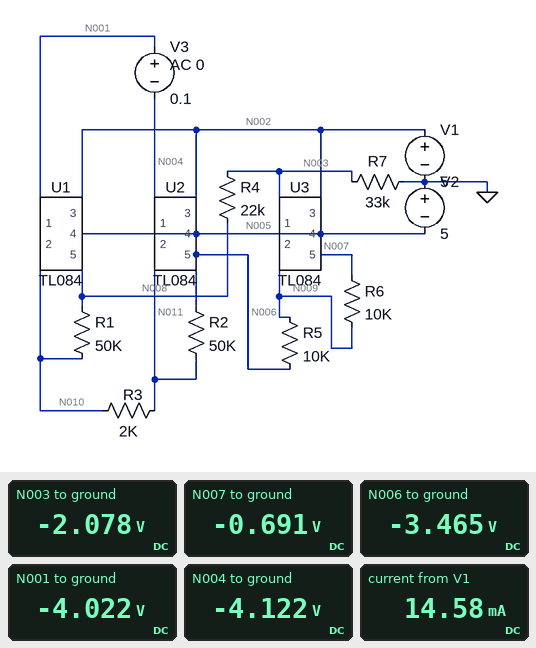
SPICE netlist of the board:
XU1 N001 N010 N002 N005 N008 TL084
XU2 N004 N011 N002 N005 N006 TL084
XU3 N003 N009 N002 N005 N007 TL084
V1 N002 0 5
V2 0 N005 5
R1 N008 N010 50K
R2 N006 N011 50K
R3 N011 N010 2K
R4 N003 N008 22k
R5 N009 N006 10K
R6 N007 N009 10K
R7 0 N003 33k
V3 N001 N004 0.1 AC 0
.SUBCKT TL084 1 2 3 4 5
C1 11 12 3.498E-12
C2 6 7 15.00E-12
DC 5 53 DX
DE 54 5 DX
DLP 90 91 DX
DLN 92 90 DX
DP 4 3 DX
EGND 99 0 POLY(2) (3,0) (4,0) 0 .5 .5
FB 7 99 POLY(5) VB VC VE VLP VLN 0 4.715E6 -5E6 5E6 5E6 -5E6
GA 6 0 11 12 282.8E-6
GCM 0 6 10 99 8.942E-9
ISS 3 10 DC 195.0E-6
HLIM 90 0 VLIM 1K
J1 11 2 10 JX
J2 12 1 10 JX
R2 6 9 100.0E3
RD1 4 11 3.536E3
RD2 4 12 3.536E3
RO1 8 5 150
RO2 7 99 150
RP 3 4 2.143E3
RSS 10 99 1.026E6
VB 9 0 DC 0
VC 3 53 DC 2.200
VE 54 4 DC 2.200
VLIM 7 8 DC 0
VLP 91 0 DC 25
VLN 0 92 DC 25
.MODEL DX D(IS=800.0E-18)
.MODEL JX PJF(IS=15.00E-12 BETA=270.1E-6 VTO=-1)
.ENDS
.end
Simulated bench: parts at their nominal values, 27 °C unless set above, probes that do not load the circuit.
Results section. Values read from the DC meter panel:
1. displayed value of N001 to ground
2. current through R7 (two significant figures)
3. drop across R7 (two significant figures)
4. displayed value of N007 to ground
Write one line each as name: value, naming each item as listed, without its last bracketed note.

displayed value of N001 to ground: -4.022 V
current through R7: 63 µA
drop across R7: 2.1 V
displayed value of N007 to ground: -0.691 V
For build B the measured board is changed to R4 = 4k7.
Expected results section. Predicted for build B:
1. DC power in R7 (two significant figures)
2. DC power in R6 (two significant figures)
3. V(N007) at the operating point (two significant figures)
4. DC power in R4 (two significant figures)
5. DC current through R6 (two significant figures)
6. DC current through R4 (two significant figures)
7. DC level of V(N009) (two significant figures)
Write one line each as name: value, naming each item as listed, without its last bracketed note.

DC power in R7: 280 µW
DC power in R6: 19 µW
V(N007) at the operating point: -2.6 V
DC power in R4: 40 µW
DC current through R6: 43 µA
DC current through R4: 92 µA
DC level of V(N009): -3.0 V
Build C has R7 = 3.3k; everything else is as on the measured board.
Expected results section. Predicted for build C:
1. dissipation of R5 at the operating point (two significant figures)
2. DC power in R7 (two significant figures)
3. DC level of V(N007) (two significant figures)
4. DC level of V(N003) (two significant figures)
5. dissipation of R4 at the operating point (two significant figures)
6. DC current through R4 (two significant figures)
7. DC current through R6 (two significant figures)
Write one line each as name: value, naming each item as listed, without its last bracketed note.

dissipation of R5 at the operating point: 910 µW
DC power in R7: 62 µW
DC level of V(N007): 2.6 V
DC level of V(N003): -450 mV
dissipation of R4 at the operating point: 410 µW
DC current through R4: 140 µA
DC current through R6: 300 µA
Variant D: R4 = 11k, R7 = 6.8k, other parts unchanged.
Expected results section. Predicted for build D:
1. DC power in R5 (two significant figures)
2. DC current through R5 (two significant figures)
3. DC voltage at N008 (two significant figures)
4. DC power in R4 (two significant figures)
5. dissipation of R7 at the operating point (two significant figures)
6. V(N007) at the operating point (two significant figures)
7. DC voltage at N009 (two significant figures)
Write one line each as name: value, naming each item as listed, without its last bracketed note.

DC power in R5: 460 µW
DC current through R5: 210 µA
DC voltage at N008: -3.5 V
DC power in R4: 420 µW
dissipation of R7 at the operating point: 260 µW
V(N007) at the operating point: 820 mV
DC voltage at N009: -1.3 V
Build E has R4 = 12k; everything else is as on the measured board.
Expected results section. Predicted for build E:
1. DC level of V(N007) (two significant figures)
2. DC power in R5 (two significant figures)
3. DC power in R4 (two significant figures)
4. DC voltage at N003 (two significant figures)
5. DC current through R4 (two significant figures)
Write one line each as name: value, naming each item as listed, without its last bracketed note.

DC level of V(N007): -1.6 V
DC power in R5: 86 µW
DC power in R4: 71 µW
DC voltage at N003: -2.5 V
DC current through R4: 77 µA
